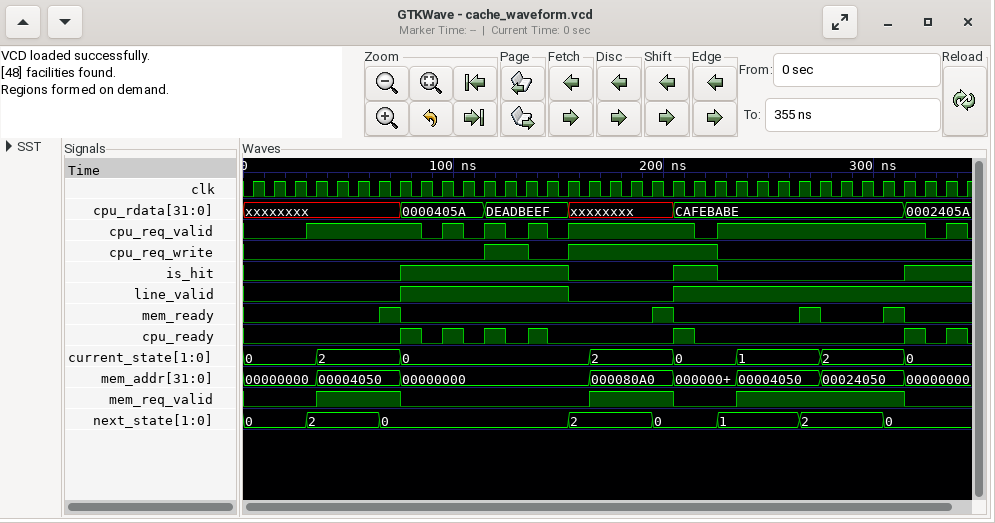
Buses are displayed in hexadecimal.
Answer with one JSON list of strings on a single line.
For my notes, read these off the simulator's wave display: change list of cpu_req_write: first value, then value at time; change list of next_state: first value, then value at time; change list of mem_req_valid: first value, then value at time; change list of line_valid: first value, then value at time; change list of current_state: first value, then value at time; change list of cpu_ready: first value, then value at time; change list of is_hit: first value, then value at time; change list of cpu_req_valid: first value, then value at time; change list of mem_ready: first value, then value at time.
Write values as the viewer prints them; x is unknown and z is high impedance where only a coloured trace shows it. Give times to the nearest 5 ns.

["0, 1 at 115 ns, 0 at 135 ns, 1 at 155 ns, 0 at 225 ns", "0, 2 at 30 ns, 0 at 65 ns, 2 at 155 ns, 0 at 195 ns, 1 at 225 ns, 2 at 265 ns, 0 at 305 ns", "0, 1 at 35 ns, 0 at 75 ns, 1 at 165 ns, 0 at 205 ns, 1 at 235 ns, 0 at 315 ns", "0, 1 at 75 ns, 0 at 155 ns, 1 at 205 ns", "0, 2 at 35 ns, 0 at 75 ns, 2 at 165 ns, 0 at 205 ns, 1 at 235 ns, 2 at 275 ns, 0 at 315 ns", "0, 1 at 75 ns, 0 at 85 ns, 1 at 95 ns, 0 at 105 ns, 1 at 115 ns, 0 at 125 ns, 1 at 135 ns, 0 at 145 ns, 1 at 205 ns, 0 at 215 ns, 1 at 315 ns, 0 at 325 ns, 1 at 335 ns, 0 at 345 ns", "0, 1 at 75 ns, 0 at 155 ns, 1 at 205 ns, 0 at 225 ns, 1 at 315 ns", "0, 1 at 30 ns, 0 at 85 ns, 1 at 95 ns, 0 at 105 ns, 1 at 115 ns, 0 at 125 ns, 1 at 135 ns, 0 at 145 ns, 1 at 155 ns, 0 at 215 ns, 1 at 225 ns, 0 at 325 ns, 1 at 335 ns, 0 at 345 ns", "0, 1 at 65 ns, 0 at 75 ns, 1 at 195 ns, 0 at 205 ns, 1 at 265 ns, 0 at 275 ns, 1 at 305 ns, 0 at 315 ns"]
